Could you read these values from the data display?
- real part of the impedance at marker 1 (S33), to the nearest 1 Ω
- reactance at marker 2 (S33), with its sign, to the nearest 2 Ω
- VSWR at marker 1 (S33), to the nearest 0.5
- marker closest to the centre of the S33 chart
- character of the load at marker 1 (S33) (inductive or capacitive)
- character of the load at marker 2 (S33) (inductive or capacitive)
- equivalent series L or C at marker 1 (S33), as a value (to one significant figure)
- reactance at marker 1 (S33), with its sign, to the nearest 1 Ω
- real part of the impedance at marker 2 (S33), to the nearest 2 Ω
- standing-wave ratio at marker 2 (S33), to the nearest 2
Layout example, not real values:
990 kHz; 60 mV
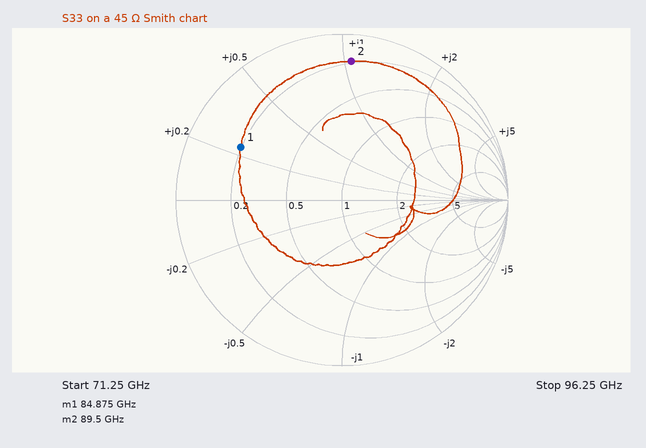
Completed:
9 Ω; +48 Ω; 5.5; marker 1; inductive; inductive; 20 pH; +11 Ω; 8 Ω; 12
